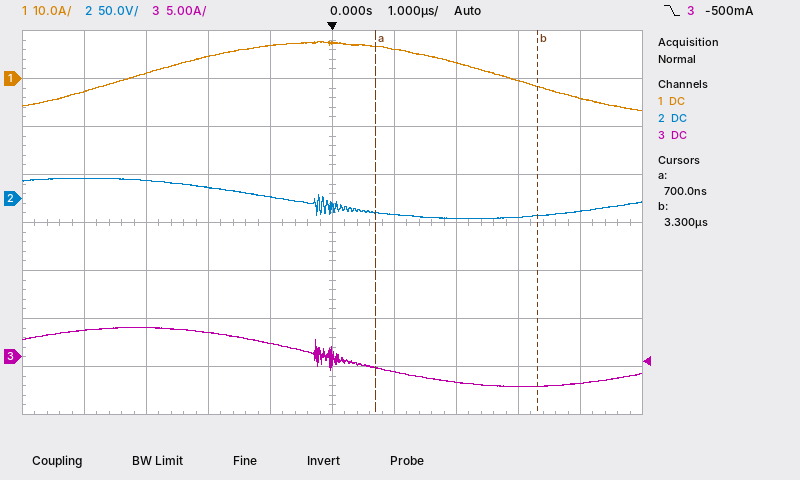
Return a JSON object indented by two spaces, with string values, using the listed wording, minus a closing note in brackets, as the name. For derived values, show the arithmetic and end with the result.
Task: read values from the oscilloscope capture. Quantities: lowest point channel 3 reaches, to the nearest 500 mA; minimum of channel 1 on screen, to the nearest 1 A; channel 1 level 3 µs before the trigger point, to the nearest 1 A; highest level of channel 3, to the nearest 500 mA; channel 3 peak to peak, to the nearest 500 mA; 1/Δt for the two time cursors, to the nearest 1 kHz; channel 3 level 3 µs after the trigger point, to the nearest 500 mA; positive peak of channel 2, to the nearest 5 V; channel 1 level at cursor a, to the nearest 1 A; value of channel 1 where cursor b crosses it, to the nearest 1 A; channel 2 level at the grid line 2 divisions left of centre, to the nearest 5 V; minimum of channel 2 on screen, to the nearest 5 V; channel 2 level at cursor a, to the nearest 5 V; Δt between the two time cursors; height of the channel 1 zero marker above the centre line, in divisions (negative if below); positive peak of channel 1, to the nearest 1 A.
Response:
{
  "lowest point channel 3 reaches, to the nearest 500 mA": "-3.0 A",
  "minimum of channel 1 on screen, to the nearest 1 A": "-7 A",
  "channel 1 level 3 µs before the trigger point, to the nearest 1 A": "1 A",
  "highest level of channel 3, to the nearest 500 mA": "3.0 A",
  "channel 3 peak to peak, to the nearest 500 mA": "3.0 A − (-3.0 A) = 6.0 A",
  "1/Δt for the two time cursors, to the nearest 1 kHz": "1 / 2.6 µs ≈ 385 kHz",
  "channel 3 level 3 µs after the trigger point, to the nearest 500 mA": "-3.0 A",
  "positive peak of channel 2, to the nearest 5 V": "20 V",
  "channel 1 level at cursor a, to the nearest 1 A": "7 A",
  "value of channel 1 where cursor b crosses it, to the nearest 1 A": "-2 A",
  "channel 2 level at the grid line 2 divisions left of centre, to the nearest 5 V": "10 V",
  "minimum of channel 2 on screen, to the nearest 5 V": "-20 V",
  "channel 2 level at cursor a, to the nearest 5 V": "-15 V",
  "Δt between the two time cursors": "3.3 µs − (700 ns) = 2.6 µs",
  "height of the channel 1 zero marker above the centre line, in divisions": "+3.0 div",
  "positive peak of channel 1, to the nearest 1 A": "8 A"
}
